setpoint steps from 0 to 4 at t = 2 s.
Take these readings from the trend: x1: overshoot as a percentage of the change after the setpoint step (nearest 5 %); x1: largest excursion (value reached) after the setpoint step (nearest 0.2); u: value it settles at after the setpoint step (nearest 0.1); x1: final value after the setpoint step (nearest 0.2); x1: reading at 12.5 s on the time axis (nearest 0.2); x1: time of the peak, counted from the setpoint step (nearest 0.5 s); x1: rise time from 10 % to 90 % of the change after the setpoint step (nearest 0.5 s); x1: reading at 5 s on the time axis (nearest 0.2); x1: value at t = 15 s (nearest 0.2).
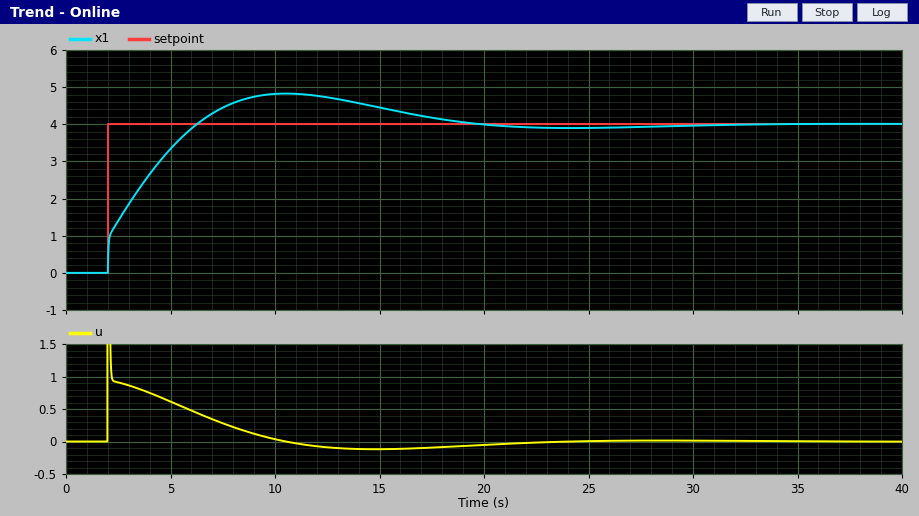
20 %
4.8
0.0
4.0
4.8
8.5 s
3.5 s
3.4
4.4
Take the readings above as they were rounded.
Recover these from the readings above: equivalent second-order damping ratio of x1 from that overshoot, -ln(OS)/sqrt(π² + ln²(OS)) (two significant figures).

0.46
